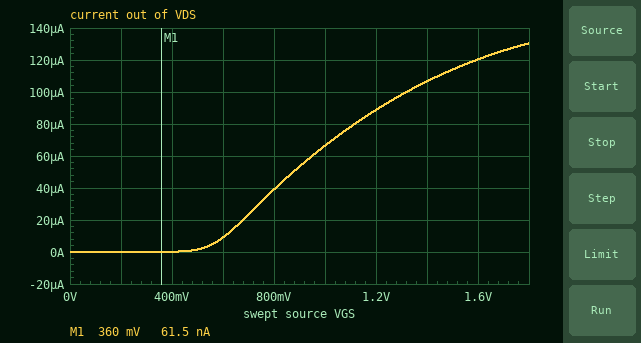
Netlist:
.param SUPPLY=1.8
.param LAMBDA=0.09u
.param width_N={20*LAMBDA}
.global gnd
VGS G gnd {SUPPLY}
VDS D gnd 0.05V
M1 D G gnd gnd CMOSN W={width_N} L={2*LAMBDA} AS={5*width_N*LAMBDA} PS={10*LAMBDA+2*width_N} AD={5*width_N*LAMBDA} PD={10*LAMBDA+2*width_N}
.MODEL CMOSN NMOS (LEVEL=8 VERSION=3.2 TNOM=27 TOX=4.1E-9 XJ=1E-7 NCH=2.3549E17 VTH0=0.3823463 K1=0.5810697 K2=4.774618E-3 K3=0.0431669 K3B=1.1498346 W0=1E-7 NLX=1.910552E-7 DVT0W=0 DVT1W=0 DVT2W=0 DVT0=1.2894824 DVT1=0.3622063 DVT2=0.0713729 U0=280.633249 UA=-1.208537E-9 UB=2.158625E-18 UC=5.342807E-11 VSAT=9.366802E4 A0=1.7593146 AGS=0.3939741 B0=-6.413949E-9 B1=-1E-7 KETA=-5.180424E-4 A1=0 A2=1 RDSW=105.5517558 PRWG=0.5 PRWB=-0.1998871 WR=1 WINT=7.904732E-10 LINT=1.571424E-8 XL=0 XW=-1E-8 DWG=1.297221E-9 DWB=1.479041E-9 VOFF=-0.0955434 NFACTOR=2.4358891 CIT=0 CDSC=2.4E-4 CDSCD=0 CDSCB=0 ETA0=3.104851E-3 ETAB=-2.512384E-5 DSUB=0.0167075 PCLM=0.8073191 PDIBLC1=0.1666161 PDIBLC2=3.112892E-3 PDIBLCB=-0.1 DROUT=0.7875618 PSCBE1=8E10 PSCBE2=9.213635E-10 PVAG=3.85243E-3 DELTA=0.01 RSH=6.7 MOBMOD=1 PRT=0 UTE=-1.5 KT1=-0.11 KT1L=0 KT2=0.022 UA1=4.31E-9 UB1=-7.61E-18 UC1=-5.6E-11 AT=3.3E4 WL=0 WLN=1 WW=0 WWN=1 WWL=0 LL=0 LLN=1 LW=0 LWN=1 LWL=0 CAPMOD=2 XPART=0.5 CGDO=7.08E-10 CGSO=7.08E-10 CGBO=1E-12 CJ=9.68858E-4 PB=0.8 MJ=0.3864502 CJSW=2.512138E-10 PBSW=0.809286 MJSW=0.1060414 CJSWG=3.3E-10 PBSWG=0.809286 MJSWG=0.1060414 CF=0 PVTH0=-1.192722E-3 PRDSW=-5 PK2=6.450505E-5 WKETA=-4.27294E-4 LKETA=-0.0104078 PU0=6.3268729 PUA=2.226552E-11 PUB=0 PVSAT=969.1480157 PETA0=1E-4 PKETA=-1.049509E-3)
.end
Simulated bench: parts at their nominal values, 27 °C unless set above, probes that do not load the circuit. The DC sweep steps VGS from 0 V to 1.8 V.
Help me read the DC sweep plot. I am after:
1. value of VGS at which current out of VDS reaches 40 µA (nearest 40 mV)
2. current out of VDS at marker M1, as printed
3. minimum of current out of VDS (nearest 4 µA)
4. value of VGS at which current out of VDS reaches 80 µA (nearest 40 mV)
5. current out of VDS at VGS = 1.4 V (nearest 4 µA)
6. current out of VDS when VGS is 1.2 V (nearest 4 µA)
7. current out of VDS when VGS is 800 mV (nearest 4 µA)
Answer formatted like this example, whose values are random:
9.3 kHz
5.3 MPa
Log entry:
800 mV
61.5 nA
0 A
1.12 V
108 µA
88 µA
40 µA
